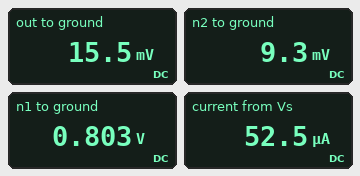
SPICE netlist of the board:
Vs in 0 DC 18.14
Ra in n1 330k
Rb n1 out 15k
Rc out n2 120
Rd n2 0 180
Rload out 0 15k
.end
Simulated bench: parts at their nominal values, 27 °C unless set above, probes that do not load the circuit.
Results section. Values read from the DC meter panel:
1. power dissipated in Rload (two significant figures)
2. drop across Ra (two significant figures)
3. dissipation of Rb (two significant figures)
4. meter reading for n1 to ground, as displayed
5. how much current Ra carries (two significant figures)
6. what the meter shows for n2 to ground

16 nW
17 V
41 µW
0.803 V
53 µA
9.3 mV
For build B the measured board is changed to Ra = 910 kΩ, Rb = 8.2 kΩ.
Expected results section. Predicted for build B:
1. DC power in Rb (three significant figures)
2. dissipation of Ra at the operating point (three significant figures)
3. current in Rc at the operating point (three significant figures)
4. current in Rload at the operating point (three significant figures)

3.20 µW
355 µW
19.4 µA
387 nA
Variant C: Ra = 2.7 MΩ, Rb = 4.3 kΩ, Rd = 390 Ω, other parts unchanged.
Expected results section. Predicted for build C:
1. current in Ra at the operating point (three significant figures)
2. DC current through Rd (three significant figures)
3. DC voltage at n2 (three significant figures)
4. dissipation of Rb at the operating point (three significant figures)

6.71 µA
6.49 µA
2.53 mV
193 nW
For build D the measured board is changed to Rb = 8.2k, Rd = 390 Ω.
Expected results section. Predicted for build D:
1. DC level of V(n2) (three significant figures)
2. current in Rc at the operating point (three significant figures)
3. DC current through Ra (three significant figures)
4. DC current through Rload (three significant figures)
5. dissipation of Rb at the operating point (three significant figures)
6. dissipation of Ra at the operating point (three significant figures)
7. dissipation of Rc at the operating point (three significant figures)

20.2 mV
51.8 µA
53.6 µA
1.76 µA
23.5 µW
947 µW
322 nW
